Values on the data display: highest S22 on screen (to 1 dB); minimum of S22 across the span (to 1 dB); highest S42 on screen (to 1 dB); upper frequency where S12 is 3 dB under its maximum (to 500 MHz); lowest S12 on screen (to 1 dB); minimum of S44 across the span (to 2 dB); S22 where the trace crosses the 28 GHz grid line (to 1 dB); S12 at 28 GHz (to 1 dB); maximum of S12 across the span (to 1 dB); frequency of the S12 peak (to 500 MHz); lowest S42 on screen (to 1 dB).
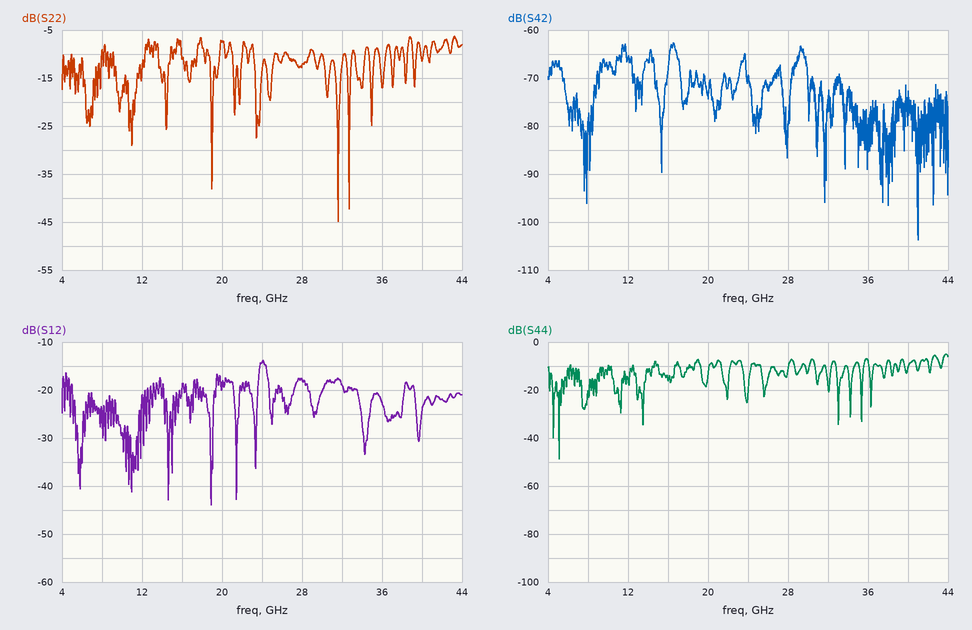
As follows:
-6 dB
-45 dB
-63 dB
24.5 GHz
-44 dB
-48 dB
-12 dB
-18 dB
-14 dB
24.0 GHz
-104 dB
